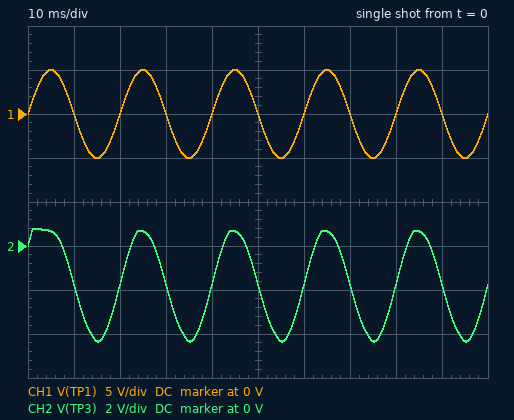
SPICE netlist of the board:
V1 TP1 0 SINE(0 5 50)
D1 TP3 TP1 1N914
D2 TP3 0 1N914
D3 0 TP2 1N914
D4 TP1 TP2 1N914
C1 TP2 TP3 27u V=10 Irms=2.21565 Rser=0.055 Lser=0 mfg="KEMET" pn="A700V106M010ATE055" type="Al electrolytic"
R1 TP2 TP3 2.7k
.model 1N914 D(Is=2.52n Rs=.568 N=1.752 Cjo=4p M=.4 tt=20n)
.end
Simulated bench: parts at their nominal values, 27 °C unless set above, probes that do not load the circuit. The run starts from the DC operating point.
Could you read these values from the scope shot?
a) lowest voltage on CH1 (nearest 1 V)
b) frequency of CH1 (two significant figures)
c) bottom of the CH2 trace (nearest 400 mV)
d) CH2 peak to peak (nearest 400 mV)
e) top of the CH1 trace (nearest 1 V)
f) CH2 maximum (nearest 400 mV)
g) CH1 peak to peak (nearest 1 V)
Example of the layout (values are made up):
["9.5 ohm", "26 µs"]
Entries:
["-5 V", "50 Hz", "-4.4 V", "5.2 V", "5 V", "800 mV", "10 V"]
